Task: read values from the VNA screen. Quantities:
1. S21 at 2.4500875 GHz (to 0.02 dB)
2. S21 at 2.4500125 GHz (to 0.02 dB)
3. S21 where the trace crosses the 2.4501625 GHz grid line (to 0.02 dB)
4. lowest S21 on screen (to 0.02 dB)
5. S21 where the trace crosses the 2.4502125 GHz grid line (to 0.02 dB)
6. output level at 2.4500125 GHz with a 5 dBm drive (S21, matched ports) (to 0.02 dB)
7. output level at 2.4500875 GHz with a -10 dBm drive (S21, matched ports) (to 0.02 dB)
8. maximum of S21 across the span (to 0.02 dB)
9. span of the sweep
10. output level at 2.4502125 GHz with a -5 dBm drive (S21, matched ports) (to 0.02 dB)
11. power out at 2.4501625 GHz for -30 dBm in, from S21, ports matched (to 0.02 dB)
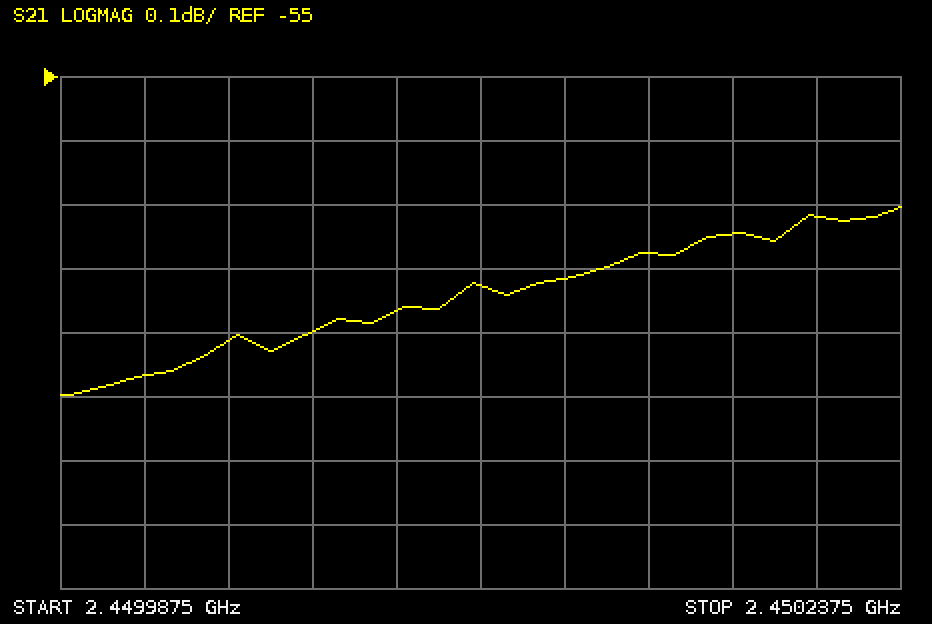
-55.36 dB
-55.46 dB
-55.28 dB
-55.50 dB
-55.22 dB
-50.46 dBm
-65.36 dBm
-55.20 dB
250 kHz
-60.22 dBm
-85.28 dBm
